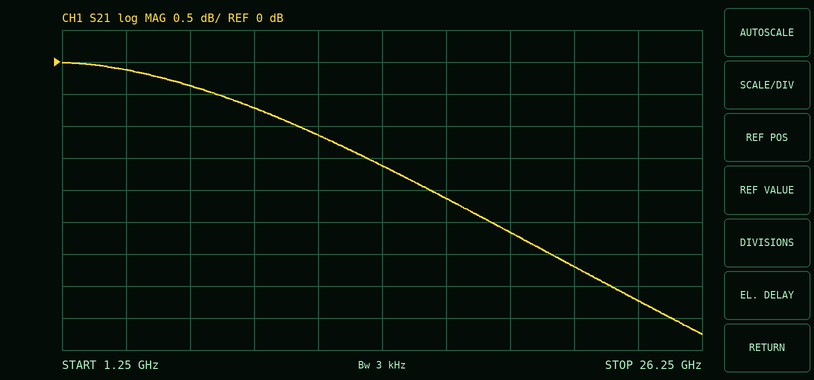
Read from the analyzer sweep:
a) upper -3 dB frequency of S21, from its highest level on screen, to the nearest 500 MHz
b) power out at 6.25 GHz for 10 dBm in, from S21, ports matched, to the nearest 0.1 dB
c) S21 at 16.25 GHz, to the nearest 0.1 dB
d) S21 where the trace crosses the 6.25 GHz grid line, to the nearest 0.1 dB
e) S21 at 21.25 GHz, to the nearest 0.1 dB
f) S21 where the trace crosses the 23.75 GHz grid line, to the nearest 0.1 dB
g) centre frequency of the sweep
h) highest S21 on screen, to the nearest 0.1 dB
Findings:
20.5 GHz
9.6 dBm
-2.1 dB
-0.4 dB
-3.2 dB
-3.7 dB
13.75 GHz
0.0 dB
